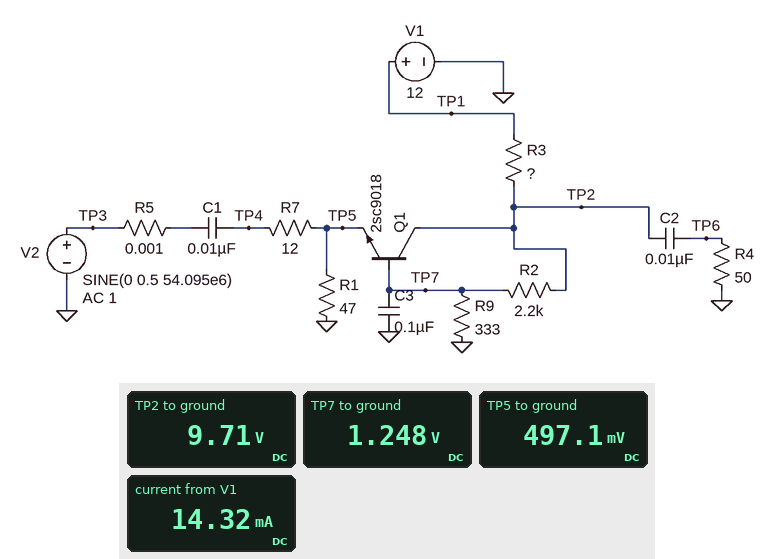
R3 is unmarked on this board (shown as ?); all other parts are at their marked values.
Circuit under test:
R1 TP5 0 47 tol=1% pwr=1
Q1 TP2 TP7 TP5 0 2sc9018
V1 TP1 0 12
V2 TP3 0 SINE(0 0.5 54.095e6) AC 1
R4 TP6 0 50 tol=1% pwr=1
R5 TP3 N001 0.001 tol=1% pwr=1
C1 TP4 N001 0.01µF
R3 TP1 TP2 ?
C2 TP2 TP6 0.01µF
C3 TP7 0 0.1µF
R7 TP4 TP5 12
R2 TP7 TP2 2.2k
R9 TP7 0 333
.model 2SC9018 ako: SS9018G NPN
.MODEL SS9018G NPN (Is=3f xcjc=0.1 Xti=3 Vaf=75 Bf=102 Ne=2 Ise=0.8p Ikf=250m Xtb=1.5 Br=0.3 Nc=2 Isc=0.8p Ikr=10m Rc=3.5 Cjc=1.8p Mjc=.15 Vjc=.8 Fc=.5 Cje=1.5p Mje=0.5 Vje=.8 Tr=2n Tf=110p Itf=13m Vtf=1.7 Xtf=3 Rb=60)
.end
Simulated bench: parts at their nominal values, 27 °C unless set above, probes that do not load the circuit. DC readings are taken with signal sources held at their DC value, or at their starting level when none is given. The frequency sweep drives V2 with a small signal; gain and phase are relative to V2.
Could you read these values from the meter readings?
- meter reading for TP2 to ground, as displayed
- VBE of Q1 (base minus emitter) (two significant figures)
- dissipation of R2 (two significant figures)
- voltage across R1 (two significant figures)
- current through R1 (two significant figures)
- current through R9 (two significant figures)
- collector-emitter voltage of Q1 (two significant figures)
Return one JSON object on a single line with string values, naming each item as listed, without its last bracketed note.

{"meter reading for TP2 to ground, as displayed": "9.71 V", "VBE of Q1 (base minus emitter)": "750 mV", "dissipation of R2": "33 mW", "voltage across R1": "500 mV", "current through R1": "11 mA", "current through R9": "3.7 mA", "collector-emitter voltage of Q1": "9.2 V"}
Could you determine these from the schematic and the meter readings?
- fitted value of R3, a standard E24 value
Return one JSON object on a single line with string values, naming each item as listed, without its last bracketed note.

{"fitted value of R3, a standard E24 value": "160 Ω"}
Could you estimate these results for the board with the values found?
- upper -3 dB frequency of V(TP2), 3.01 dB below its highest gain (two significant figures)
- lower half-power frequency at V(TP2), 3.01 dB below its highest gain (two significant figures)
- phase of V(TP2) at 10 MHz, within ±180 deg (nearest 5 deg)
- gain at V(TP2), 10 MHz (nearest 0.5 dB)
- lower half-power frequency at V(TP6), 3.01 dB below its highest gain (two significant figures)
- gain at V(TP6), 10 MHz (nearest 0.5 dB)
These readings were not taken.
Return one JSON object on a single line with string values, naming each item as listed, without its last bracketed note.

{"upper -3 dB frequency of V(TP2), 3.01 dB below its highest gain": "230 MHz", "lower half-power frequency at V(TP2), 3.01 dB below its highest gain": "970 kHz", "phase of V(TP2) at 10 MHz, within ±180 deg": "0 deg", "gain at V(TP2), 10 MHz": "7.5 dB", "lower half-power frequency at V(TP6), 3.01 dB below its highest gain": "1.1 MHz", "gain at V(TP6), 10 MHz": "7.5 dB"}
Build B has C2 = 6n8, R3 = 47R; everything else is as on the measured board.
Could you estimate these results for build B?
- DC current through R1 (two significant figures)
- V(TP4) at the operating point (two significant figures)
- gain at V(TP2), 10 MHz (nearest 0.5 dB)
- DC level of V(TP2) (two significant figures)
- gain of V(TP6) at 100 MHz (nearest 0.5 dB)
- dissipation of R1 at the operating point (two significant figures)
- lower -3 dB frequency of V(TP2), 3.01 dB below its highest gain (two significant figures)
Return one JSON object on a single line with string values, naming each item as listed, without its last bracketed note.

{"DC current through R1": "14 mA", "V(TP4) at the operating point": "670 mV", "gain at V(TP2), 10 MHz": "4.0 dB", "DC level of V(TP2)": "11 V", "gain of V(TP6) at 100 MHz": "3.0 dB", "dissipation of R1 at the operating point": "9.4 mW", "lower -3 dB frequency of V(TP2), 3.01 dB below its highest gain": "960 kHz"}
